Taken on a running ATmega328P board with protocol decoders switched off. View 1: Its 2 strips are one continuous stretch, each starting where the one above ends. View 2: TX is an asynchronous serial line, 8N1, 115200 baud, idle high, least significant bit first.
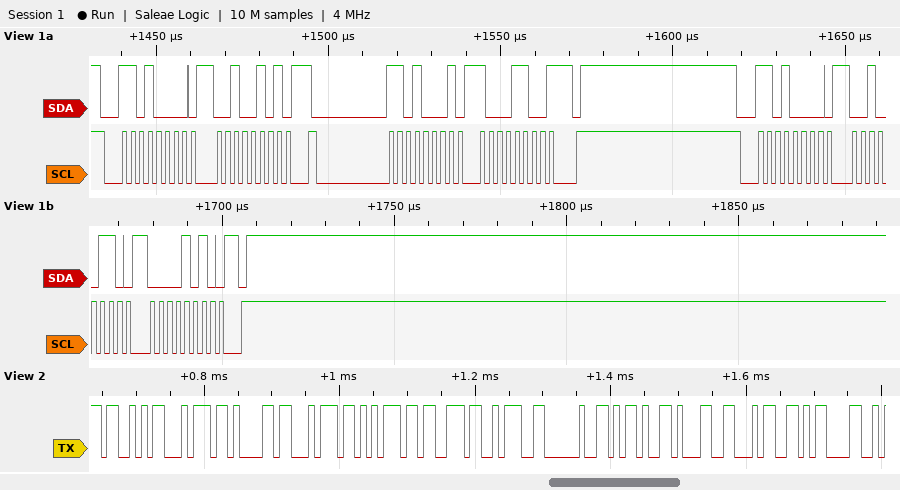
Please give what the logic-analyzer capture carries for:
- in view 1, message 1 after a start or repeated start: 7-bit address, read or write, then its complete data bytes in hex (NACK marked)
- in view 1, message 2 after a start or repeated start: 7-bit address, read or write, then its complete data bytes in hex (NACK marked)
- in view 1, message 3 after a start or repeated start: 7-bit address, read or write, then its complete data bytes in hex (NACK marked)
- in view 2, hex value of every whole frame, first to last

0x68 write: 25
0x68 read: 8C NACK
0x68 write: 26 0A
53 74 61 74 75 73 3A 20 2D 31 34 0D
